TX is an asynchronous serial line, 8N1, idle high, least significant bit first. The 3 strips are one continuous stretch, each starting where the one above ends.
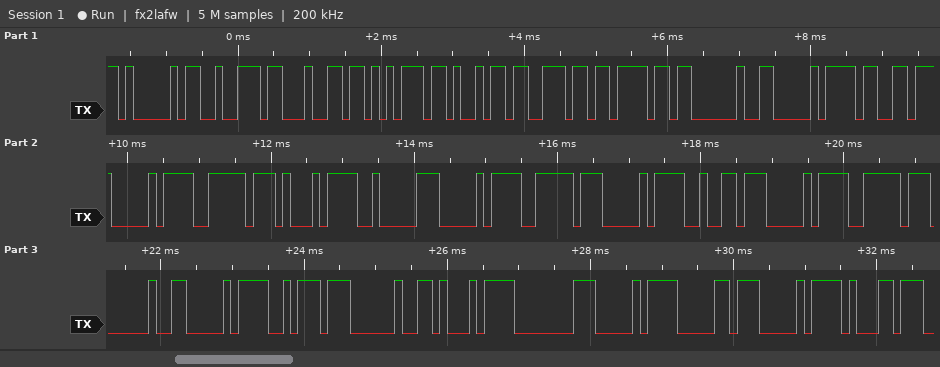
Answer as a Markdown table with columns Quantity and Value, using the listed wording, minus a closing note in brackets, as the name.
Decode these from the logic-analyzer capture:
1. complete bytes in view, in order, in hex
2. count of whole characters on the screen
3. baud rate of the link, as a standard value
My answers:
| Quantity | Value |
|---|---|
| complete bytes in view, in order, in hex | 0x41 0x72 0x64 0x75 0x69 0x6E 0x6F 0x20 0xD0 0xB3 0xD0 0xBE 0xD1 0x82 0xD0 0xBE 0xD0 0xB2 0xD0 0xBE 0x20 0xD0 0xBA 0x20 0xD1 0x80 0xD0 0xB0 0xD0 0xB1 |
| count of whole characters on the screen | 30 |
| baud rate of the link, as a standard value | 9600 baud |
